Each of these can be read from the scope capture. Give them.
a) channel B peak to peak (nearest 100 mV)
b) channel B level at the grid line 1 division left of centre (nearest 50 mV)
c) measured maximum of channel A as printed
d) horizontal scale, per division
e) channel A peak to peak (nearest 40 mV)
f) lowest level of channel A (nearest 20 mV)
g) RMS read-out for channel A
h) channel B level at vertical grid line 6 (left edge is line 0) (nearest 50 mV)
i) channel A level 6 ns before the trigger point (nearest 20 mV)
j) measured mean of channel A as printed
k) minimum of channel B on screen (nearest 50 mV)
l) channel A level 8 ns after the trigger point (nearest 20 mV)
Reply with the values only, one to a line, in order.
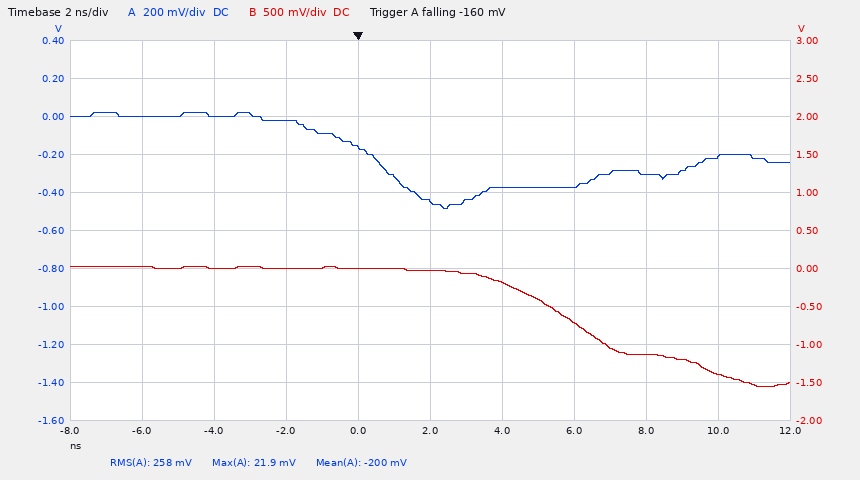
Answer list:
1.60 V
0 mV
21.9 mV
2 ns
520 mV
-480 mV
258 mV
-200 mV
0 mV
-200 mV
-1.55 V
-300 mV
